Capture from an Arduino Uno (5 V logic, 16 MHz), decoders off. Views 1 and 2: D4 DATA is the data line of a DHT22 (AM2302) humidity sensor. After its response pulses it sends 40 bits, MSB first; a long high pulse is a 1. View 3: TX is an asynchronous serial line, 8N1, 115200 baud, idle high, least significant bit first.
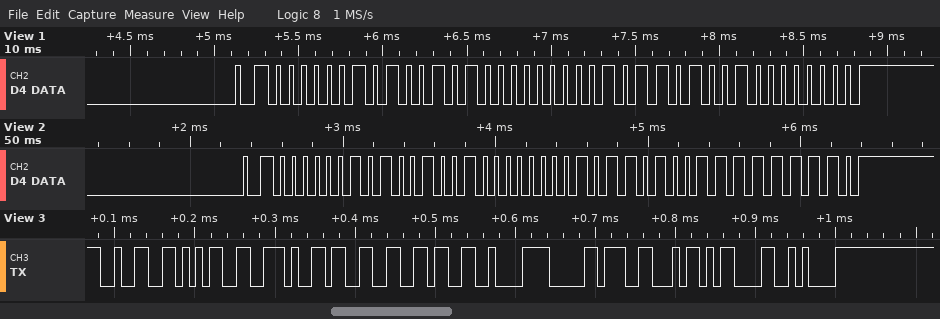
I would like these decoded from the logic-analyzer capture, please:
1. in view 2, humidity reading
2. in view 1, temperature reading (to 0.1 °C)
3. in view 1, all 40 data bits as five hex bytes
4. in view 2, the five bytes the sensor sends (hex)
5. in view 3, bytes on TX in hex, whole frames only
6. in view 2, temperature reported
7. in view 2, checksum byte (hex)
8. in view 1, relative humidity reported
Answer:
65.8 %
36.1 °C
02 94 01 69 00
02 92 01 69 FE
32 35 2E 33 36 C2 B0 46 0D 0A
36.1 °C
0xFE
66.0 %
